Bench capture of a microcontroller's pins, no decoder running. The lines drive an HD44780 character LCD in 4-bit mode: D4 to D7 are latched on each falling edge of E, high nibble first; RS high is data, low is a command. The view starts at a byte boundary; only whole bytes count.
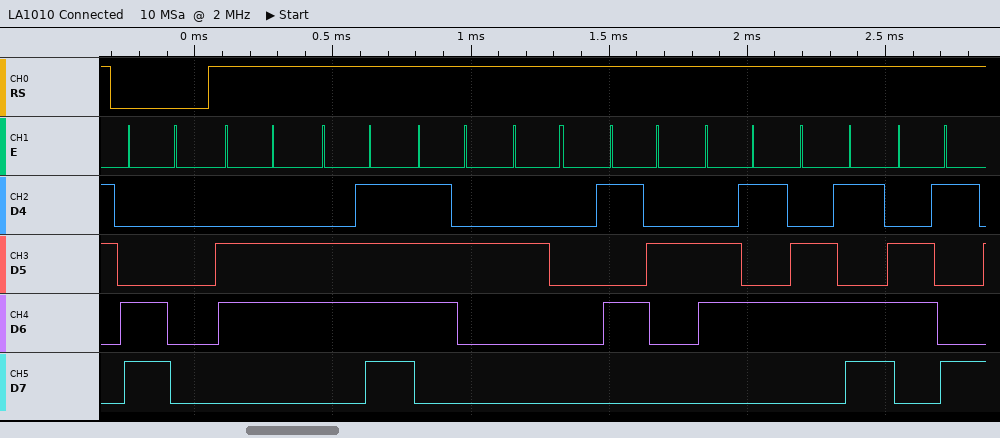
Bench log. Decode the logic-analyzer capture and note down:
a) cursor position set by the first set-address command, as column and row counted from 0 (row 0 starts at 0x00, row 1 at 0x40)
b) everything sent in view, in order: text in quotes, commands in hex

column 0, row 1
0xC0 "for Remi"
